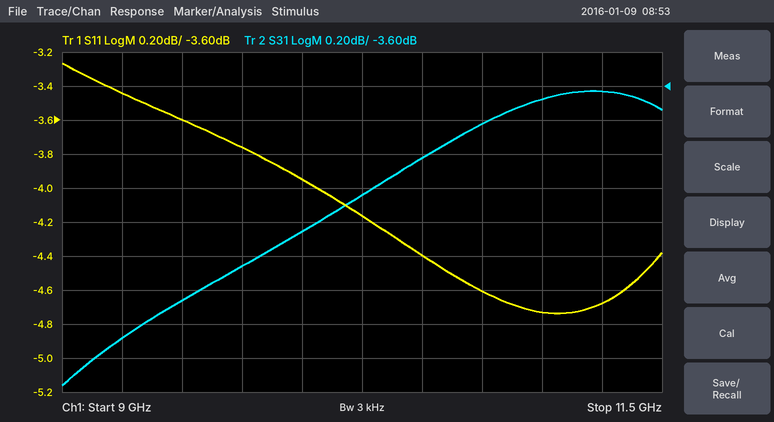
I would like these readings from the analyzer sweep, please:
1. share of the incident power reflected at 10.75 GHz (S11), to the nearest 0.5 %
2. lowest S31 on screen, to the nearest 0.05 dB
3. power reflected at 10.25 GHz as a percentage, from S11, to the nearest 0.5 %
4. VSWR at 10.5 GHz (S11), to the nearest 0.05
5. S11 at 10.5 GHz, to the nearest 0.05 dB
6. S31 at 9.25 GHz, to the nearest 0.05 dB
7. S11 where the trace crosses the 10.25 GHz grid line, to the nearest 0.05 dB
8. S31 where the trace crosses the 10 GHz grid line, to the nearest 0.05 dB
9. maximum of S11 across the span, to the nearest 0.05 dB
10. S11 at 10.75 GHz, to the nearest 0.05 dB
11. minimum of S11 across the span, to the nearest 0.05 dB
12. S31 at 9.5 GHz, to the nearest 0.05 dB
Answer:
34.5 %
-5.35 dB
38.5 %
4.05
-4.40 dB
-5.10 dB
-4.15 dB
-4.45 dB
-3.25 dB
-4.60 dB
-4.75 dB
-4.85 dB
